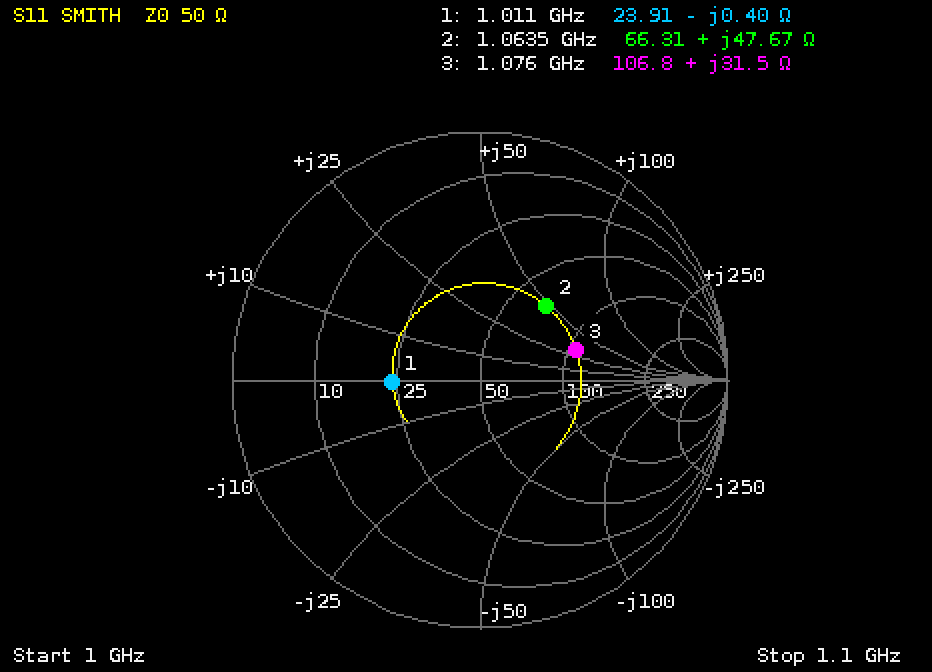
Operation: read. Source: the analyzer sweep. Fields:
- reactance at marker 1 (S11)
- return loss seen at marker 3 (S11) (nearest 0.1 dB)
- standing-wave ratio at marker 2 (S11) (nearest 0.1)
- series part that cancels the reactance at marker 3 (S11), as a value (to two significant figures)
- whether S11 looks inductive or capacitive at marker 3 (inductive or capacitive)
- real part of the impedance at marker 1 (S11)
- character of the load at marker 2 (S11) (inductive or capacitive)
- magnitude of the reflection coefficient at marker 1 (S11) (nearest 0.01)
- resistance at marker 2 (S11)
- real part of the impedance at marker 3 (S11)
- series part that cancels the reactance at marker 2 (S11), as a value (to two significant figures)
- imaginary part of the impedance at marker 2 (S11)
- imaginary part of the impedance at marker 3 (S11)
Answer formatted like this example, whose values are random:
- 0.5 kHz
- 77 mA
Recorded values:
- -0.40 Ω
- 7.8 dB
- 2.3
- 4.7 pF
- inductive
- 23.91 Ω
- inductive
- 0.35
- 66.31 Ω
- 106.8 Ω
- 3.1 pF
- +47.67 Ω
- +31.5 Ω
